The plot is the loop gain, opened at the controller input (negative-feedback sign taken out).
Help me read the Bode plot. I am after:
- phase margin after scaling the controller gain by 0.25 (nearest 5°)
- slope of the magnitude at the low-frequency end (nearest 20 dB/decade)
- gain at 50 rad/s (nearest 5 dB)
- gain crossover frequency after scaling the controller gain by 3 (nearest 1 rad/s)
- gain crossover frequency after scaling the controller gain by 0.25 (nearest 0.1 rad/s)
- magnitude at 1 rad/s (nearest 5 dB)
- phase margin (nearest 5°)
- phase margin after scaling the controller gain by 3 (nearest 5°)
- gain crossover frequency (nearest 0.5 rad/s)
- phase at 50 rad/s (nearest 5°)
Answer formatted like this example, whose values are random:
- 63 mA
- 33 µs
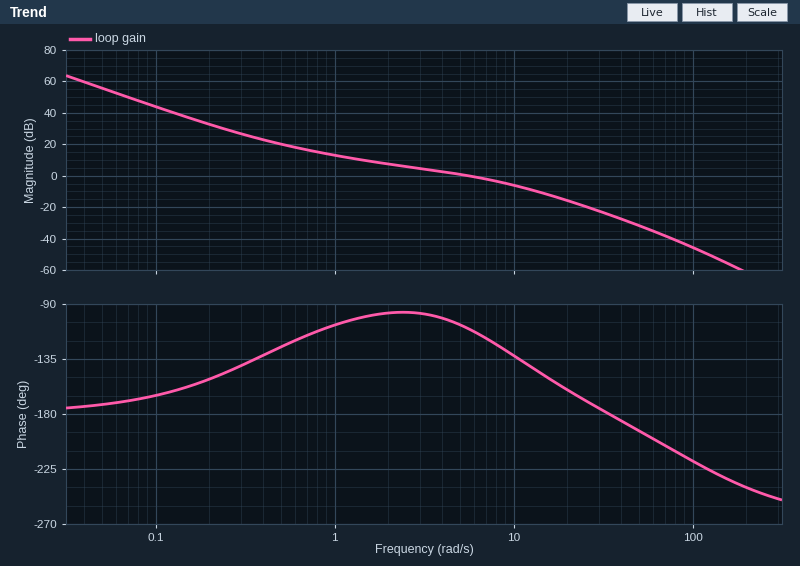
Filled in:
- 75°
- -40 dB/decade
- -30 dB
- 13 rad/s
- 1.1 rad/s
- 15 dB
- 70°
- 35°
- 5.5 rad/s
- -195°
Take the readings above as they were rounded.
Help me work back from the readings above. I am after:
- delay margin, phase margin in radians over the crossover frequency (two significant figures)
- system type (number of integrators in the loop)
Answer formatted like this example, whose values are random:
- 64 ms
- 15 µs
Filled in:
- 0.22 s
- 2
